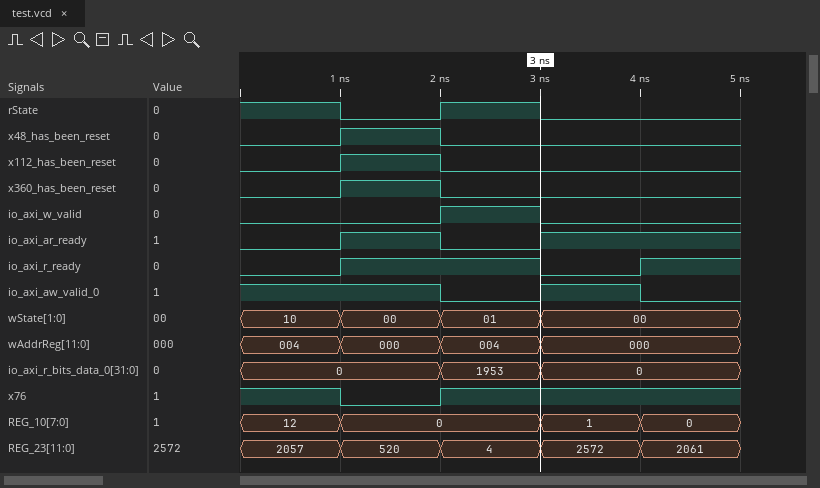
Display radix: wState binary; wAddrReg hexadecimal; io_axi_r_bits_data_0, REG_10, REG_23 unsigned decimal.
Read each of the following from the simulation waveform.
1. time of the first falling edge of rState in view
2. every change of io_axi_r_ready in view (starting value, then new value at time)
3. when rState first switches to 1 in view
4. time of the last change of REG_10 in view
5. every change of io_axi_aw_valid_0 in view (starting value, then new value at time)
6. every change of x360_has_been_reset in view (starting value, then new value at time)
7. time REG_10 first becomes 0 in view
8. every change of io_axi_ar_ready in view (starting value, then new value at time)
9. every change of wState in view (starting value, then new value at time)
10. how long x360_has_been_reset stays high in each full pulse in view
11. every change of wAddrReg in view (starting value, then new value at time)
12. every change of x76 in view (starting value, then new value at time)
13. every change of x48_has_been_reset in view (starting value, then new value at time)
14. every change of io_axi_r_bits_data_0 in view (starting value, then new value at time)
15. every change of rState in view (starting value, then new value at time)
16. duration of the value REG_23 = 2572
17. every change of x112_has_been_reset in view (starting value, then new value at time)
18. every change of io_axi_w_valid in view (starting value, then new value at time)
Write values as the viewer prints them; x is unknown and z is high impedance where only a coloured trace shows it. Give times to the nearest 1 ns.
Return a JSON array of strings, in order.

["1 ns", "0, 1 at 1 ns, 0 at 3 ns, 1 at 4 ns", "2 ns", "4 ns", "1, 0 at 2 ns, 1 at 3 ns, 0 at 4 ns", "0, 1 at 1 ns, 0 at 2 ns", "1 ns", "0, 1 at 1 ns, 0 at 2 ns, 1 at 3 ns", "10, 00 at 1 ns, 01 at 2 ns, 00 at 3 ns", "1 ns", "004, 000 at 1 ns, 004 at 2 ns, 000 at 3 ns", "1, 0 at 1 ns, 1 at 2 ns", "0, 1 at 1 ns, 0 at 2 ns", "0, 1953 at 2 ns, 0 at 3 ns", "1, 0 at 1 ns, 1 at 2 ns, 0 at 3 ns", "1 ns", "0, 1 at 1 ns, 0 at 2 ns", "0, 1 at 2 ns, 0 at 3 ns"]
